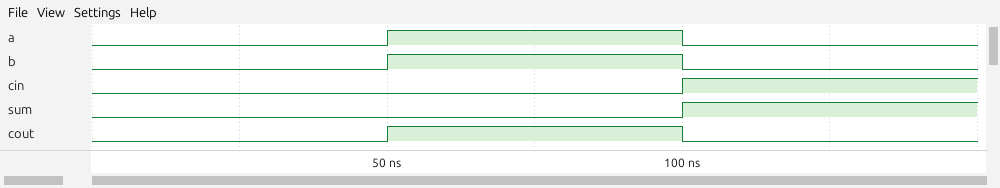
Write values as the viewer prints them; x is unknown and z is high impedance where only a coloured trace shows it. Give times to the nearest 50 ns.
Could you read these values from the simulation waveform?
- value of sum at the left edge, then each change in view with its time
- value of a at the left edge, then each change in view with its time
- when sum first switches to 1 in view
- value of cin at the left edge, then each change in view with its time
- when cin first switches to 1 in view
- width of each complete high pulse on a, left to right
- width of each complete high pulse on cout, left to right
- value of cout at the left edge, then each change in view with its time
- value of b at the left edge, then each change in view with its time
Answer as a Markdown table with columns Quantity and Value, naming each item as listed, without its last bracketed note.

| Quantity | Value |
|---|---|
| value of sum at the left edge, then each change in view with its time | 0, 1 at 100 ns |
| value of a at the left edge, then each change in view with its time | 0, 1 at 50 ns, 0 at 100 ns |
| when sum first switches to 1 in view | 100 ns |
| value of cin at the left edge, then each change in view with its time | 0, 1 at 100 ns |
| when cin first switches to 1 in view | 100 ns |
| width of each complete high pulse on a, left to right | 50 ns |
| width of each complete high pulse on cout, left to right | 50 ns |
| value of cout at the left edge, then each change in view with its time | 0, 1 at 50 ns, 0 at 100 ns |
| value of b at the left edge, then each change in view with its time | 0, 1 at 50 ns, 0 at 100 ns |
